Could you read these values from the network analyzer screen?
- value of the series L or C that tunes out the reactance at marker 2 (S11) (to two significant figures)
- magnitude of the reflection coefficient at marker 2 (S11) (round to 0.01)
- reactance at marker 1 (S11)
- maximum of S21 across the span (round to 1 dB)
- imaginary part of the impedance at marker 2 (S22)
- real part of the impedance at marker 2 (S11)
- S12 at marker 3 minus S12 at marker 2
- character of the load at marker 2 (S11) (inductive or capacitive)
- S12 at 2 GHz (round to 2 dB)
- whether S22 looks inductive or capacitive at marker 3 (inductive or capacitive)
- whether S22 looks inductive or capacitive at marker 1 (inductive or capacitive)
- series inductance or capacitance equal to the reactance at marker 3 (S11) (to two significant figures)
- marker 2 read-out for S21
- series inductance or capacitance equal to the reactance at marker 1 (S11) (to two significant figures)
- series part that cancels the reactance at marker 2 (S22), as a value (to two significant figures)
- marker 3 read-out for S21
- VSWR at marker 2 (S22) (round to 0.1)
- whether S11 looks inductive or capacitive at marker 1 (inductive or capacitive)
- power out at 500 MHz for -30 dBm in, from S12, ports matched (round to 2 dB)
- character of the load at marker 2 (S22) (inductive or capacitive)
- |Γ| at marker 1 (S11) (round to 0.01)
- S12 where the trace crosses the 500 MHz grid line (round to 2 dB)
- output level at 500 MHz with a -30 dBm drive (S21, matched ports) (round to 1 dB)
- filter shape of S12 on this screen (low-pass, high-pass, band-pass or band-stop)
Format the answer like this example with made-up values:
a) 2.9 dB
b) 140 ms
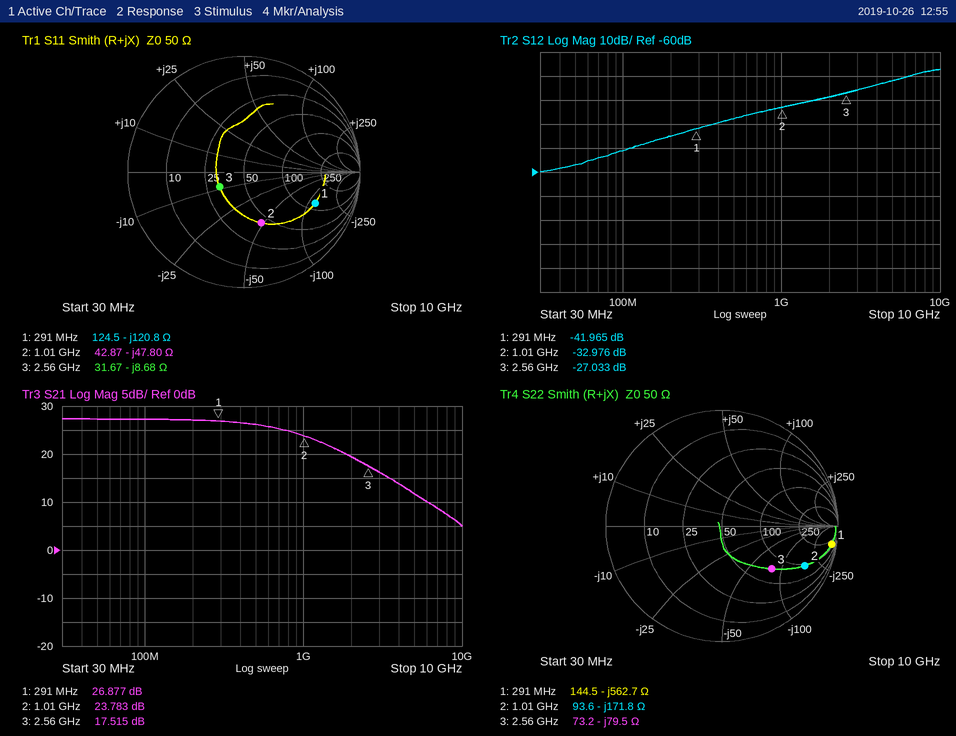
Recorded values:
a) 7.5 nH
b) 0.46
c) -120.8 Ω
d) 27 dB
e) -171.8 Ω
f) 42.87 Ω
g) 5.943 dB
h) capacitive
i) -28 dB
j) capacitive
k) capacitive
l) 7.2 pF
m) 23.783 dB
n) 4.5 pF
o) 27 nH
p) 17.515 dB
q) 8.6
r) capacitive
s) -68 dBm
t) capacitive
u) 0.67
v) -38 dB
w) -4 dBm
x) high-pass
